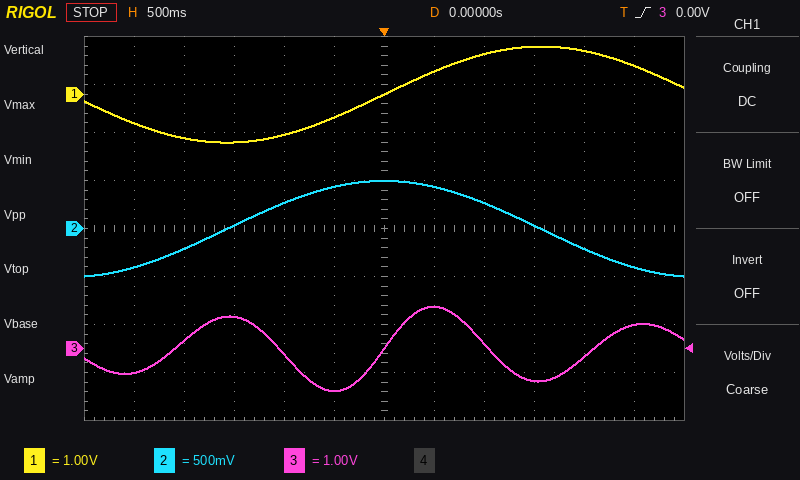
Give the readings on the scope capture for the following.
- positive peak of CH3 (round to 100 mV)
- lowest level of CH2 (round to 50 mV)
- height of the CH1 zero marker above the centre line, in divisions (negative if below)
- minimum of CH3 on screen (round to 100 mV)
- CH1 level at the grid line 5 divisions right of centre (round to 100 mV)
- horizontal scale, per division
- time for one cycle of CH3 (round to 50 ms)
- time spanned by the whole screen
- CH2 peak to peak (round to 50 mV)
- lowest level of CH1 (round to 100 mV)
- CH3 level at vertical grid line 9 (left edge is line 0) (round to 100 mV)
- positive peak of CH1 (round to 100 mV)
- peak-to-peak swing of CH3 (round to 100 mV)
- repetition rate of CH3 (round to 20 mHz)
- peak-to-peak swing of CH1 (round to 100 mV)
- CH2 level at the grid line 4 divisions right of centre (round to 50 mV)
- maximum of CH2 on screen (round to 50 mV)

900 mV
-500 mV
+2.8 div
-900 mV
600 mV
500 ms
2.10 s
6 s
1.00 V
-1.0 V
-700 mV
1.0 V
1.8 V
480 mHz
2.0 V
-200 mV
500 mV
